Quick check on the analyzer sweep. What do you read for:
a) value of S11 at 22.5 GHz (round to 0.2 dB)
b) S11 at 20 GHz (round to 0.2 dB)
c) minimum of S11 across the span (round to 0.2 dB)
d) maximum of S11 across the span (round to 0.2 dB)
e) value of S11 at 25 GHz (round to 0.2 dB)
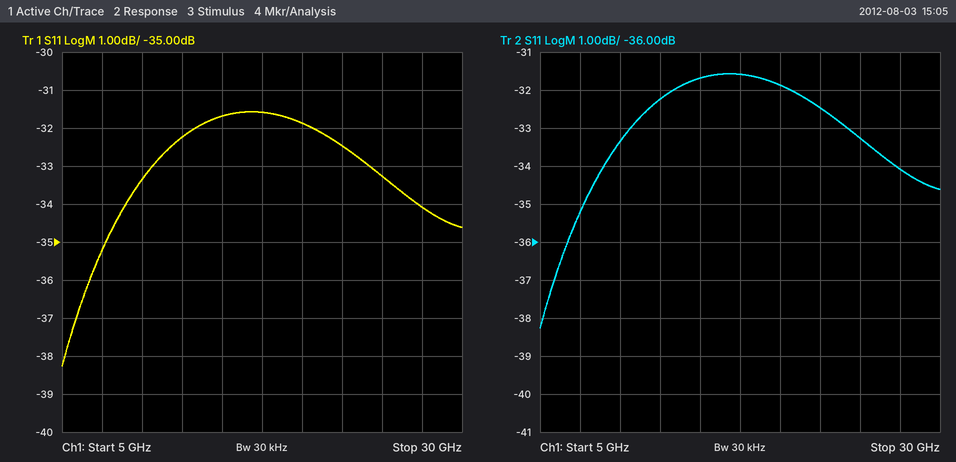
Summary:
-32.4 dB
-31.8 dB
-38.2 dB
-31.6 dB
-33.2 dB
